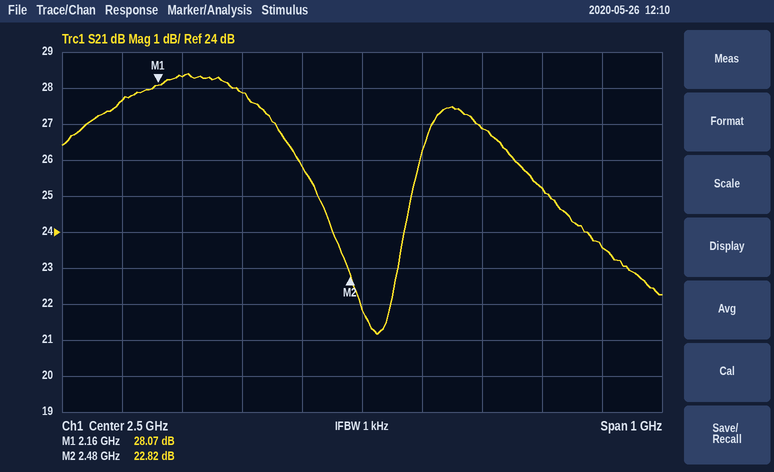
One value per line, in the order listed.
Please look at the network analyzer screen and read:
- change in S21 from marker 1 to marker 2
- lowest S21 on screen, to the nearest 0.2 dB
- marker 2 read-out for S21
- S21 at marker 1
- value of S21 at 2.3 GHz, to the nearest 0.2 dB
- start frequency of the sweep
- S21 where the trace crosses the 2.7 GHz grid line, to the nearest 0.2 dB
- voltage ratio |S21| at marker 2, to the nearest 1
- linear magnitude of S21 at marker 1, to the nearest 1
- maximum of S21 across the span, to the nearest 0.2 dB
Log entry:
-5.25 dB
21.2 dB
22.82 dB
28.07 dB
27.8 dB
2 GHz
26.8 dB
14
25
28.4 dB
